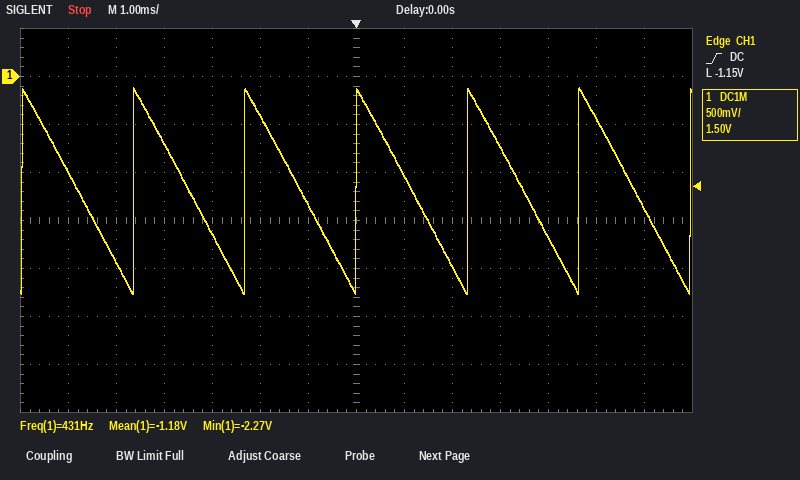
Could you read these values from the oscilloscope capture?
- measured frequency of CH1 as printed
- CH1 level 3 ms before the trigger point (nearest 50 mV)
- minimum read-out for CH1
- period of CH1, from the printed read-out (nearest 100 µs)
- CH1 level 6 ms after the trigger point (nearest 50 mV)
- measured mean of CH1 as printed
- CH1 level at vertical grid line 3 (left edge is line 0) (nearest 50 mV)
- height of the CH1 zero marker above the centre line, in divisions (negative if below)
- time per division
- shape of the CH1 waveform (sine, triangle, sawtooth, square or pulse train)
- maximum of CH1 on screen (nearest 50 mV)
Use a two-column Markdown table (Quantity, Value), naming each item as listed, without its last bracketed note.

| Quantity | Value |
|---|---|
| measured frequency of CH1 as printed | 431 Hz |
| CH1 level 3 ms before the trigger point | -1.65 V |
| minimum read-out for CH1 | -2.27 V |
| period of CH1, from the printed read-out | 2.3 ms |
| CH1 level 6 ms after the trigger point | -1.35 V |
| measured mean of CH1 as printed | -1.18 V |
| CH1 level at vertical grid line 3 (left edge is line 0) | -700 mV |
| height of the CH1 zero marker above the centre line, in divisions | +3.0 div |
| time per division | 1 ms |
| shape of the CH1 waveform | sawtooth |
| maximum of CH1 on screen | -100 mV |
